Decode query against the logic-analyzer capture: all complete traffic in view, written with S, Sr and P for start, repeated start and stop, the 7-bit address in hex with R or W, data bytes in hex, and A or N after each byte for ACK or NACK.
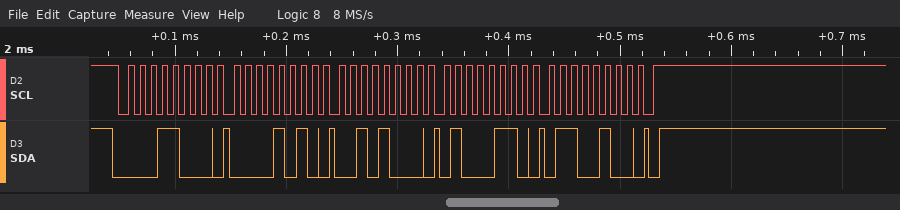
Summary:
S 0CW A 0A A 28 A 46 A 64 A P
